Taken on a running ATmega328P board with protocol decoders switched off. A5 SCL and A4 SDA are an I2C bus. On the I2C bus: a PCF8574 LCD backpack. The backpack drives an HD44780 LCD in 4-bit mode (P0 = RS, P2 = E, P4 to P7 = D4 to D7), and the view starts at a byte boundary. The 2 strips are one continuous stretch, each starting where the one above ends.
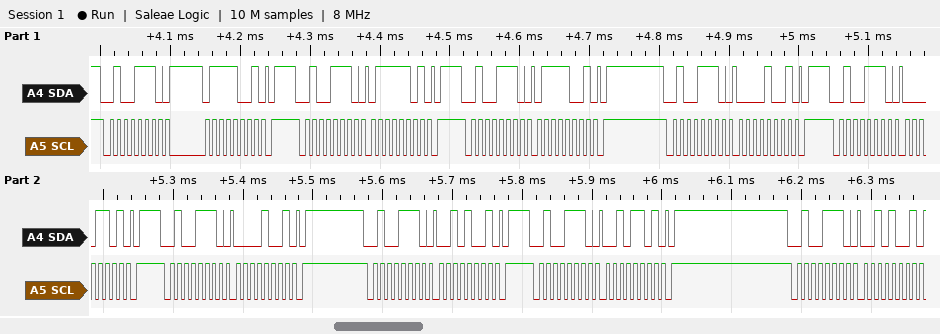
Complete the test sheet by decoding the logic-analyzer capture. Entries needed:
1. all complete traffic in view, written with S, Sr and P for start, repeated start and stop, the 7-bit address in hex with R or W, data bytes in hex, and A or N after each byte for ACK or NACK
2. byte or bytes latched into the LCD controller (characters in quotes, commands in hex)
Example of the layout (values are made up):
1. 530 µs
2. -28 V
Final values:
1. S 27W A 79 A P S 27W A 7D A P S 27W A 79 A P S 27W A 09 A P S 27W A 0D A P S 27W A 09 A P S 27W A 29 A P S 27W A 2D A P S 27W A 29 A
2. 'p'
